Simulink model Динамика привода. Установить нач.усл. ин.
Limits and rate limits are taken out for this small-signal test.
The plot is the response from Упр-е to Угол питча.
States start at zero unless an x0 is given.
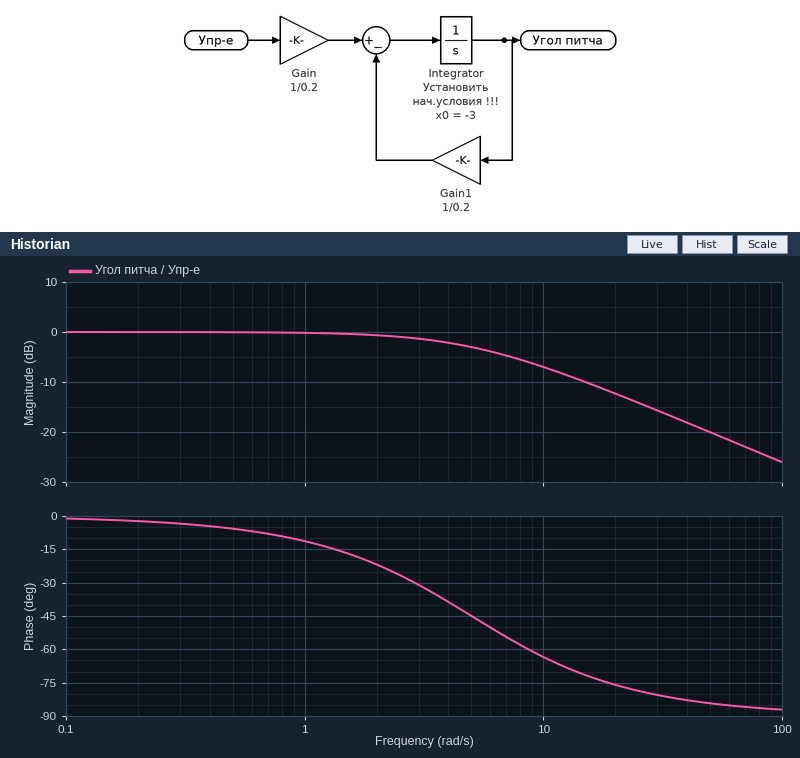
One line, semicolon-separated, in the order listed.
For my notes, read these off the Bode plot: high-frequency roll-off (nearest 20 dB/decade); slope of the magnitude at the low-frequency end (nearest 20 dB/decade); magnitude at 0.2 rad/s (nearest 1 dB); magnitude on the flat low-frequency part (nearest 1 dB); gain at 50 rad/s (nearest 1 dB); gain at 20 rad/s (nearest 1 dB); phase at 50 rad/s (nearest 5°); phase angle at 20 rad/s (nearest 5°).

-20 dB/decade; 0 dB/decade; 0 dB; 0 dB; -20 dB; -12 dB; -85°; -75°
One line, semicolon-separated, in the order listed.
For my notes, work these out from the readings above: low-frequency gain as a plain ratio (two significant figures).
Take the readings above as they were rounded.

1.0
